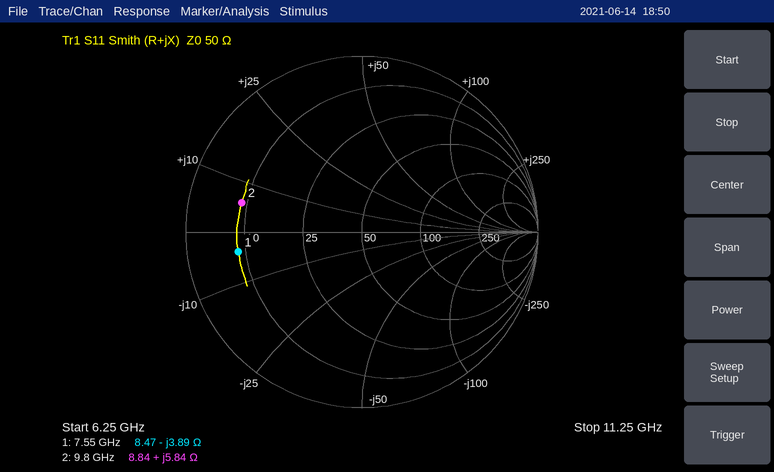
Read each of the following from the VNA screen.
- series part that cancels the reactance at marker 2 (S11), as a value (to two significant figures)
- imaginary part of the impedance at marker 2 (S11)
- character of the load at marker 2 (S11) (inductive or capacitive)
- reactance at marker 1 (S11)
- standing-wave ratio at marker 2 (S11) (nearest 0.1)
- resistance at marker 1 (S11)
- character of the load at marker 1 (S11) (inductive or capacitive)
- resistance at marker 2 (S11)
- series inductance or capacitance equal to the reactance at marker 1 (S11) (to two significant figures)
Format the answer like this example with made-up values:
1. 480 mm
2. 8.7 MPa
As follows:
1. 2.8 pF
2. +5.84 Ω
3. inductive
4. -3.89 Ω
5. 5.7
6. 8.47 Ω
7. capacitive
8. 8.84 Ω
9. 5.4 pF
